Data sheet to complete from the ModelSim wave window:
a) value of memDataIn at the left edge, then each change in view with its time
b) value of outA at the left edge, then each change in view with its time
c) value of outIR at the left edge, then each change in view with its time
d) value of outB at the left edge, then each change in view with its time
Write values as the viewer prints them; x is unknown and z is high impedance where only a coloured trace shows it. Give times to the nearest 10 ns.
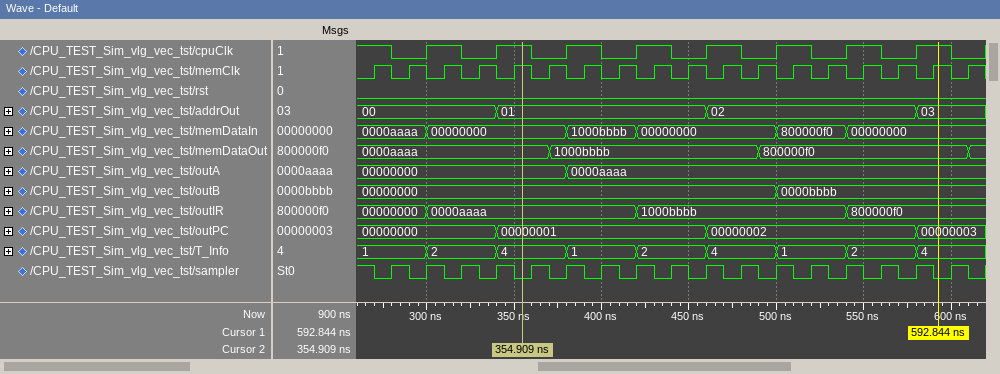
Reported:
0000aaaa, 00000000 at 300 ns, 1000bbbb at 380 ns, 00000000 at 420 ns, 800000f0 at 500 ns, 00000000 at 540 ns
00000000, 0000aaaa at 380 ns
00000000, 0000aaaa at 300 ns, 1000bbbb at 420 ns, 800000f0 at 540 ns
00000000, 0000bbbb at 500 ns
